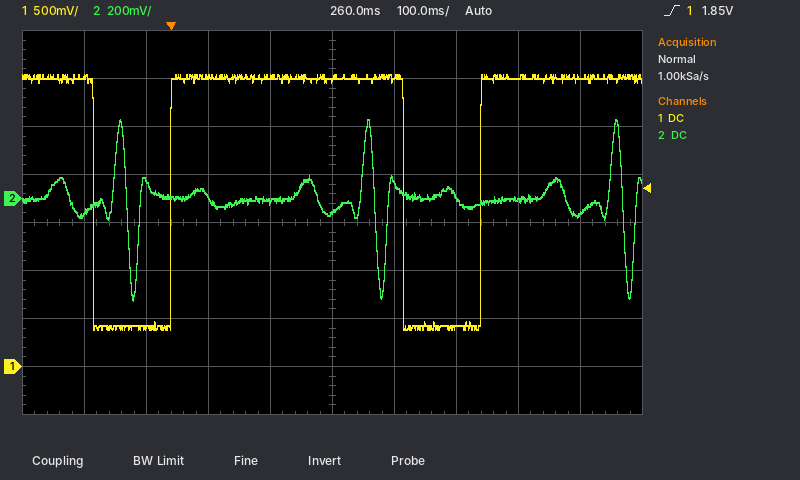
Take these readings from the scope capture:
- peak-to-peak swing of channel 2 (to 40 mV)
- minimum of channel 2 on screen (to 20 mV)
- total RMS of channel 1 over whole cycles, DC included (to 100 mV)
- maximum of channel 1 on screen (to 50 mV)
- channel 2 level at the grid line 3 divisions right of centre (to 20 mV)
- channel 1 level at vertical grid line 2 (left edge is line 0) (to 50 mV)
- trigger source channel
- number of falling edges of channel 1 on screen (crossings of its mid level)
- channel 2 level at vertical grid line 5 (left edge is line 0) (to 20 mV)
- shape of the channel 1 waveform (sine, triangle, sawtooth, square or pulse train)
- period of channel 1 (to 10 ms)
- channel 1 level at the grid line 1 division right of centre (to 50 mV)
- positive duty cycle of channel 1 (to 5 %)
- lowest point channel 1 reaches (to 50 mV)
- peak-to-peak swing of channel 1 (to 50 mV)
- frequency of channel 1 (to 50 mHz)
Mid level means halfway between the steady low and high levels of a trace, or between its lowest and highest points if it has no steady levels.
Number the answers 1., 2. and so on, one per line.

1. 760 mV
2. -420 mV
3. 2.6 V
4. 3.05 V
5. 0 mV
6. 400 mV
7. channel 1
8. 2
9. -60 mV
10. pulse train
11. 500 ms
12. 3.00 V
13. 75 %
14. 400 mV
15. 2.65 V
16. 2.00 Hz
